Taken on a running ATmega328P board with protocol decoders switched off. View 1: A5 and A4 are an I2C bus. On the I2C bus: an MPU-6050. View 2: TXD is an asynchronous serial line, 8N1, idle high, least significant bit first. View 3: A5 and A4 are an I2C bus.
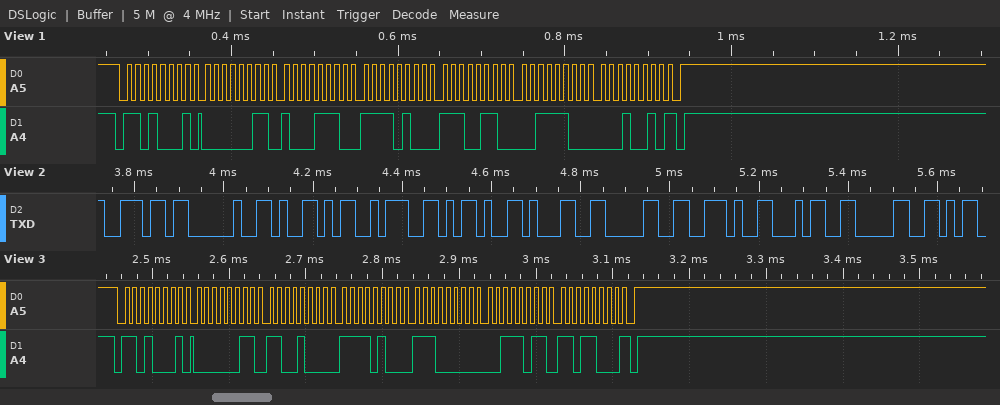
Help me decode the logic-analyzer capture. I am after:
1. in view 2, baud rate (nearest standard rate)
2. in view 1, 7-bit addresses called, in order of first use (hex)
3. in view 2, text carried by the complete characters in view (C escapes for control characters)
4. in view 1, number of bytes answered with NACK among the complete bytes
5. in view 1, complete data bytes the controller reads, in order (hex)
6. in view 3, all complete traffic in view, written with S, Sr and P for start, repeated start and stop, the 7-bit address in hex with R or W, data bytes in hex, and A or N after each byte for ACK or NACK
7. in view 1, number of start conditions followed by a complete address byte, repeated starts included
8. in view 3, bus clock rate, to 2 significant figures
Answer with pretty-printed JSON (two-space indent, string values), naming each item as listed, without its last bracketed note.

{
  "in view 2, baud rate": "57600 baud",
  "in view 1, 7-bit addresses called, in order of first use": "0x68",
  "in view 2, text carried by the complete characters in view": "\"n Y:-10.40\"",
  "in view 1, number of bytes answered with NACK among the complete bytes": "1",
  "in view 1, complete data bytes the controller reads, in order": "03 8E F4 E6 3C 12",
  "in view 3, all complete traffic in view, written with S, Sr and P for start, repeated start and stop, the 7-bit address in hex with R or W, data bytes in hex, and A or N after each byte for ACK or NACK": "S 68R A 03 A C8 A F4 A E0 A 3B A D8 N P",
  "in view 1, number of start conditions followed by a complete address byte, repeated starts included": "1",
  "in view 3, bus clock rate, to 2 significant figures": "100 kHz"
}
